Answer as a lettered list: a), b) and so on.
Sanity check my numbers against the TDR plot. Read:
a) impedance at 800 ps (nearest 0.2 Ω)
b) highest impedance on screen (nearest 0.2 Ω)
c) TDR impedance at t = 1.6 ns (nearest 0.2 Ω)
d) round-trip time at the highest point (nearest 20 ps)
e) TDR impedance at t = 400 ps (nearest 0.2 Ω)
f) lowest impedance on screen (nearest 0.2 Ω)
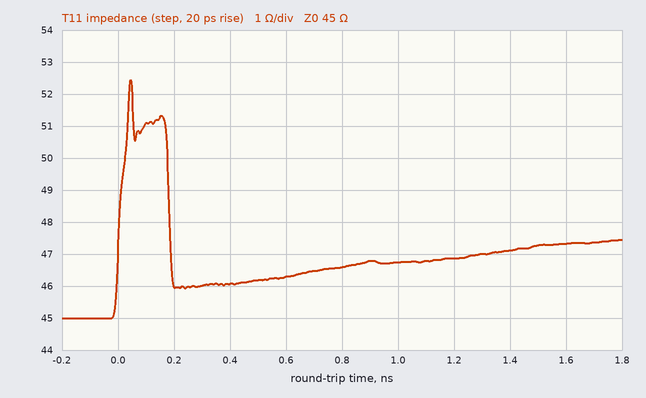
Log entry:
a) 46.6 Ω
b) 52.4 Ω
c) 47.4 Ω
d) 40 ps
e) 46.0 Ω
f) 45.0 Ω
